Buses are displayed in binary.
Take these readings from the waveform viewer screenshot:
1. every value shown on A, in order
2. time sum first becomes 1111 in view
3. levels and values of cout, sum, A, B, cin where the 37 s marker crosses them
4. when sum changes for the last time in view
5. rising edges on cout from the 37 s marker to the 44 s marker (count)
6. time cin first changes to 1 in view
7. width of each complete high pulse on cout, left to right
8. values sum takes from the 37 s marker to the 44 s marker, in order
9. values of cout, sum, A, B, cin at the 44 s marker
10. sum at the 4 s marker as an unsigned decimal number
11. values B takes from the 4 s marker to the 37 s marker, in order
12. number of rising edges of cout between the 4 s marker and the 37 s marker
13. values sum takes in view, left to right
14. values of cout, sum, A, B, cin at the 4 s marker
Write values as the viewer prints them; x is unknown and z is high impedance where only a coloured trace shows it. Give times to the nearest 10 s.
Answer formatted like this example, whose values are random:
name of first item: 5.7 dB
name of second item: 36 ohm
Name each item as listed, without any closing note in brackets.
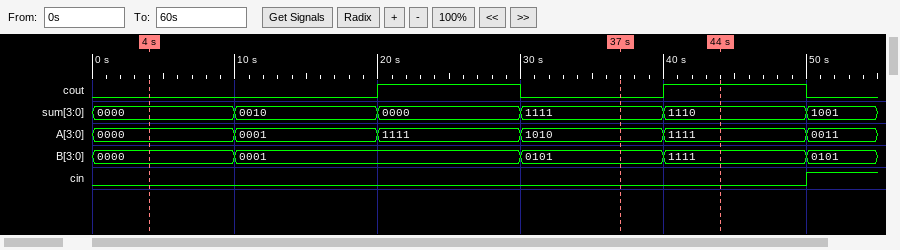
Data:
every value shown on A, in order: 0000, 0001, 1111, 1010, 1111, 0011
time sum first becomes 1111 in view: 30 s
levels and values of cout, sum, A, B, cin where the 37 s marker crosses them: cout=0, sum=1111, A=1010, B=0101, cin=0
when sum changes for the last time in view: 50 s
rising edges on cout from the 37 s marker to the 44 s marker: 1
time cin first changes to 1 in view: 50 s
width of each complete high pulse on cout, left to right: 10 s, 10 s
values sum takes from the 37 s marker to the 44 s marker, in order: 1111, 1110
values of cout, sum, A, B, cin at the 44 s marker: cout=1, sum=1110, A=1111, B=1111, cin=0
sum at the 4 s marker as an unsigned decimal number: 0
values B takes from the 4 s marker to the 37 s marker, in order: 0000, 0001, 0101
number of rising edges of cout between the 4 s marker and the 37 s marker: 1
values sum takes in view, left to right: 0000, 0010, 0000, 1111, 1110, 1001
values of cout, sum, A, B, cin at the 4 s marker: cout=0, sum=0000, A=0000, B=0000, cin=0
